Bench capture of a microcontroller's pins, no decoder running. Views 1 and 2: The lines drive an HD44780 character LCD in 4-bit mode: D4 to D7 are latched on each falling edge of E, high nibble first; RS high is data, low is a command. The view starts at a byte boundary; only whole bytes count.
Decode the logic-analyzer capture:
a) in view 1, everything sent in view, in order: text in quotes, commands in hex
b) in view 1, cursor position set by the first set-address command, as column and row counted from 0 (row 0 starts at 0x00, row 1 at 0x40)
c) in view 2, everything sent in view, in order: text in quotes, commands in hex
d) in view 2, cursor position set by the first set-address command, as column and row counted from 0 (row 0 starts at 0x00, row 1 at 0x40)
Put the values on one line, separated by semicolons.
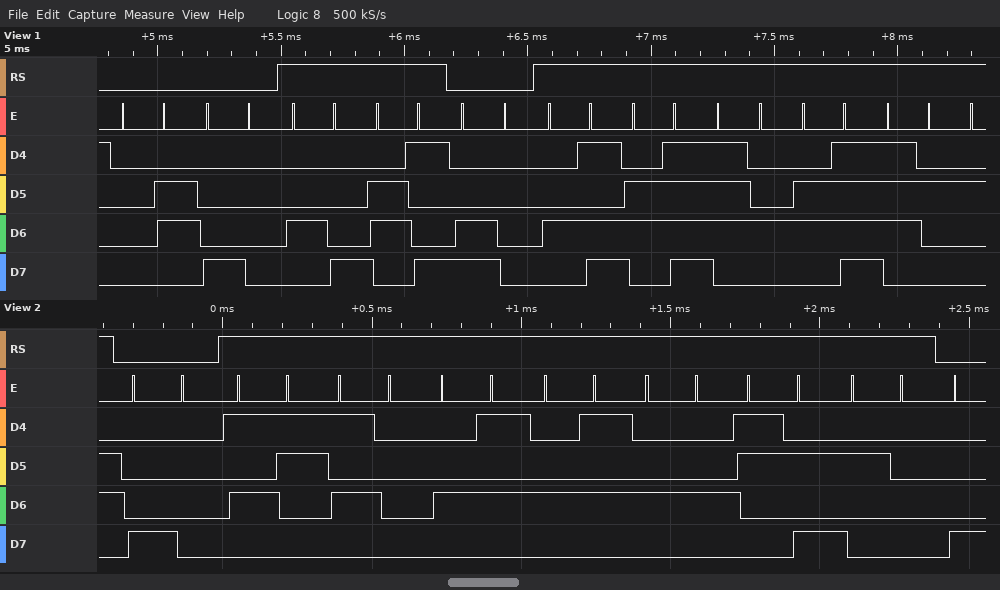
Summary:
0x06 0x80 "Hi" 0xC0 "Motor"; column 0, row 0; 0x80 "SPEED: "; column 0, row 0
